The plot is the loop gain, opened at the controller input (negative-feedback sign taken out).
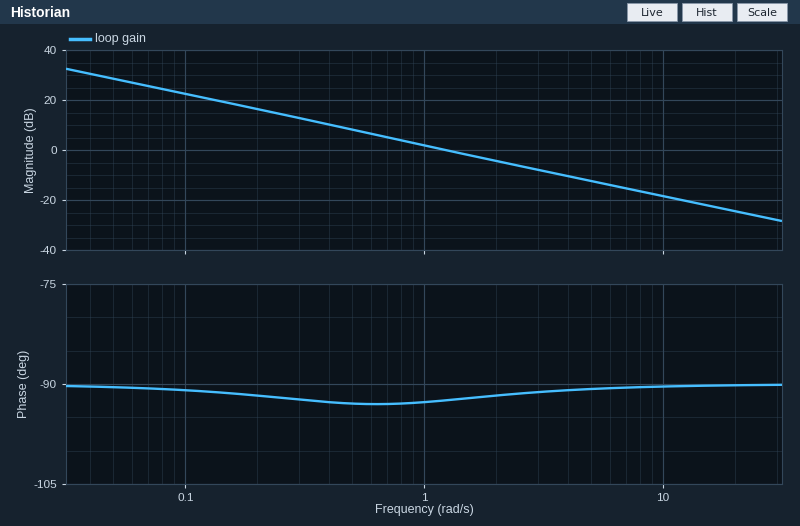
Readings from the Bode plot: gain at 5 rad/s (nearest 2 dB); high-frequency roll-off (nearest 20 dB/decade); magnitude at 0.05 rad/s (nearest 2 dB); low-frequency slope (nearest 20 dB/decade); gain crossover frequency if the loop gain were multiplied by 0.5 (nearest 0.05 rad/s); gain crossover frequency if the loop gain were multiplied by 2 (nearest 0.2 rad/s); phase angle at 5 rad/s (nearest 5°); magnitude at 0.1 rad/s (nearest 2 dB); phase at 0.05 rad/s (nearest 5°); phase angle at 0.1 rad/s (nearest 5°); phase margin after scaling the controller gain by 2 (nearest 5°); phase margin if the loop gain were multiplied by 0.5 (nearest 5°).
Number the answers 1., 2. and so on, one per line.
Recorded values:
1. -12 dB
2. -20 dB/decade
3. 28 dB
4. -20 dB/decade
5. 0.65 rad/s
6. 2.4 rad/s
7. -90°
8. 22 dB
9. -90°
10. -90°
11. 90°
12. 85°
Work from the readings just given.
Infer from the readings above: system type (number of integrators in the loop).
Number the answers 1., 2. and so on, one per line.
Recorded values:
1. 1
